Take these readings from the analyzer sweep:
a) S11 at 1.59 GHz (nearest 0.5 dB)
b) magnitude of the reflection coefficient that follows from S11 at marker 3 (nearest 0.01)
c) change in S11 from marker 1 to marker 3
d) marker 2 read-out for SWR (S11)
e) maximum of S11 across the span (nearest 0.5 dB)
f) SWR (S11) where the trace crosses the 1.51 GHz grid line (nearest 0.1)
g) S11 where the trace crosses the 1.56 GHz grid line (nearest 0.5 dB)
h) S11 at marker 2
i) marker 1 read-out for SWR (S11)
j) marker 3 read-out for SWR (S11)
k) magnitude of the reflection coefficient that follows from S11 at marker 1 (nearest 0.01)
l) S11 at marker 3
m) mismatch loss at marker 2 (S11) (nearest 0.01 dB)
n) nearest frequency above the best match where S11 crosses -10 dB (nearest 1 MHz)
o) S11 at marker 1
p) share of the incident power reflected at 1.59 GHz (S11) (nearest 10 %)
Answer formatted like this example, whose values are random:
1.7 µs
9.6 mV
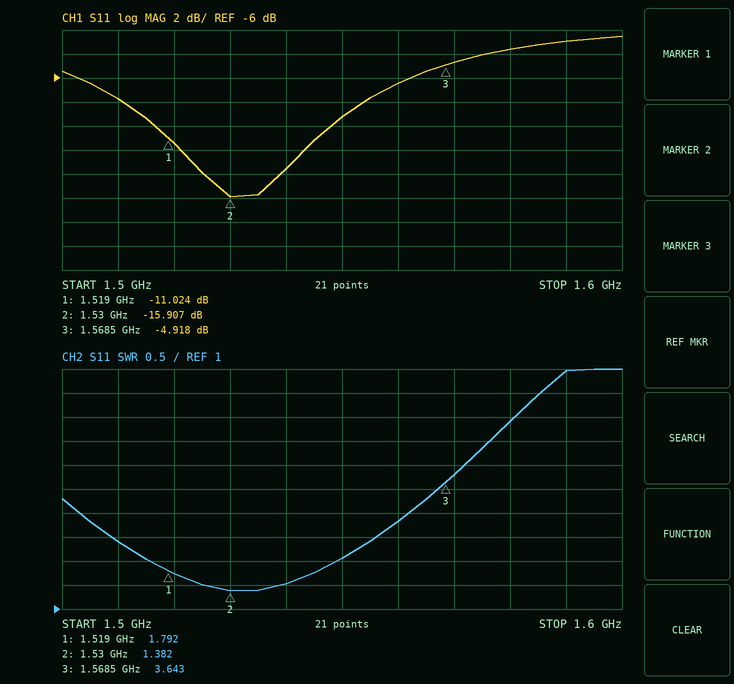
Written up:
-3.0 dB
0.57
6.106 dB
1.382
-2.5 dB
2.4
-6.5 dB
-15.907 dB
1.792
3.643
0.28
-4.918 dB
0.11 dB
1.548 GHz
-11.024 dB
50 %
